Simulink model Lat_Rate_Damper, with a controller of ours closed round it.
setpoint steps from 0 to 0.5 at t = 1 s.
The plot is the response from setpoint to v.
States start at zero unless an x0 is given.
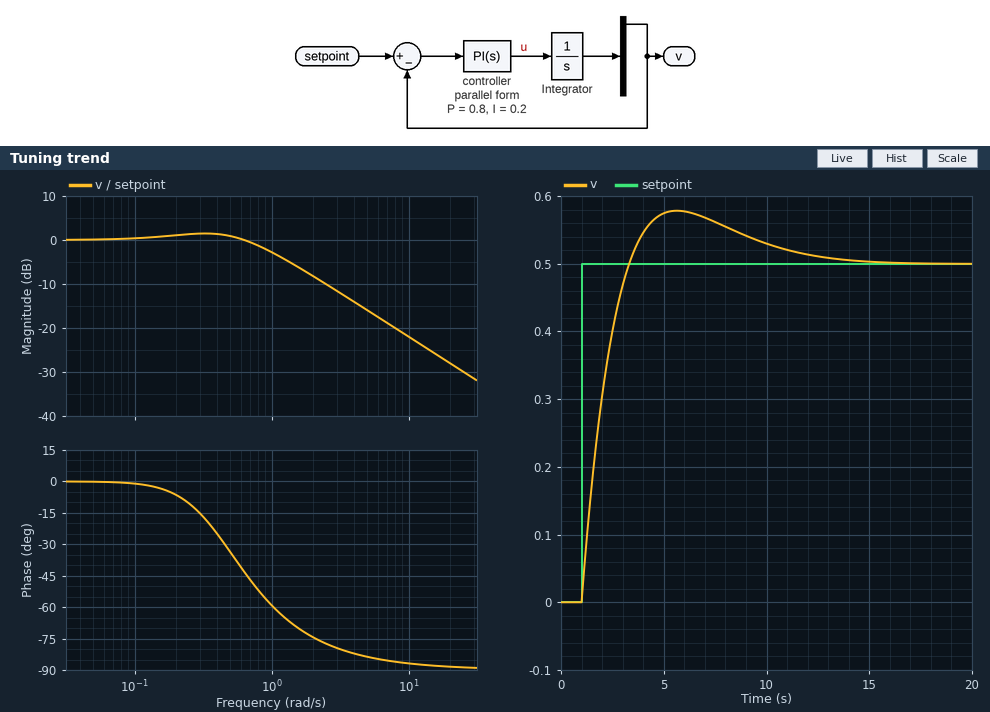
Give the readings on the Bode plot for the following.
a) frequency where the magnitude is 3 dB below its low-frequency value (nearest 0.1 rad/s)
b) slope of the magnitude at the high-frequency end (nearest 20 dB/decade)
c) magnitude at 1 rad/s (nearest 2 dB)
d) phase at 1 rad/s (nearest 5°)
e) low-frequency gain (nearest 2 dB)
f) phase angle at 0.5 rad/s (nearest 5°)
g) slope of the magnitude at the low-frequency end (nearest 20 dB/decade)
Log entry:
1.0 rad/s
-20 dB/decade
-2 dB
-60°
0 dB
-35°
0 dB/decade
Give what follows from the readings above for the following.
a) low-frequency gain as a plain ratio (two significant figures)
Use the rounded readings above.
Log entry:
1.0
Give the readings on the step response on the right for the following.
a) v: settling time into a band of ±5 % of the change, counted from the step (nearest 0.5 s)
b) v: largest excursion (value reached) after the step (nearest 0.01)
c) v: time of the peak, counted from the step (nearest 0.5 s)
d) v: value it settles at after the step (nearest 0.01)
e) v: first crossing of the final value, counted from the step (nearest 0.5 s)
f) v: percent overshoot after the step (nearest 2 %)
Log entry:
9.5 s
0.58
4.5 s
0.50
2.5 s
16 %
